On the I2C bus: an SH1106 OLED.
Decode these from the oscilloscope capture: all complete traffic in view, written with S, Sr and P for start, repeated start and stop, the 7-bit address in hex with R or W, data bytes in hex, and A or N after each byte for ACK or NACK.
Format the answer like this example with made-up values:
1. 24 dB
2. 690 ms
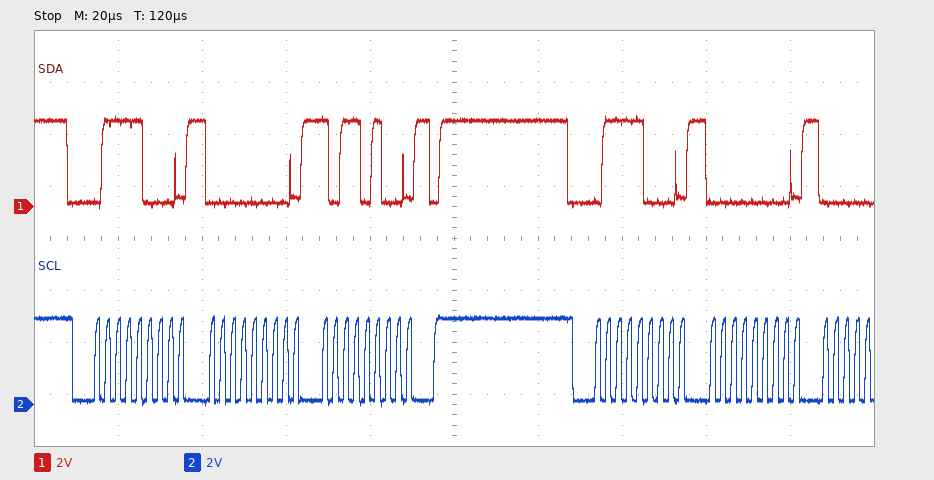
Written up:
1. S 3CW A 00 A B4 A P S 3CW A 00 A
